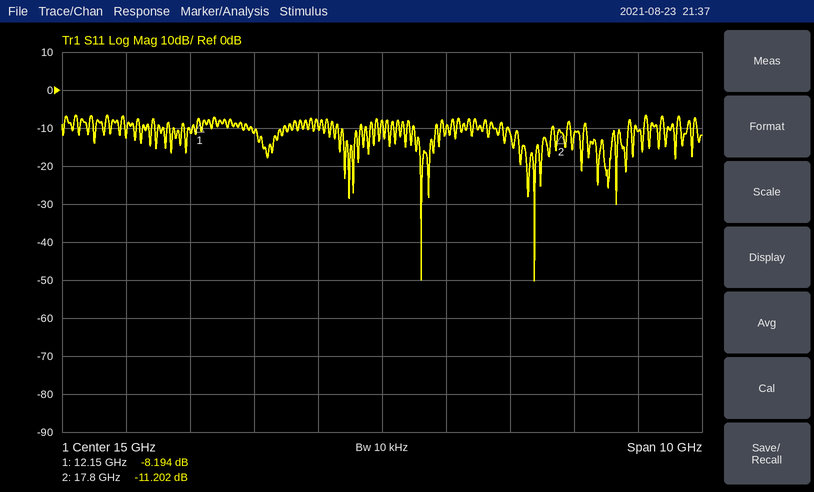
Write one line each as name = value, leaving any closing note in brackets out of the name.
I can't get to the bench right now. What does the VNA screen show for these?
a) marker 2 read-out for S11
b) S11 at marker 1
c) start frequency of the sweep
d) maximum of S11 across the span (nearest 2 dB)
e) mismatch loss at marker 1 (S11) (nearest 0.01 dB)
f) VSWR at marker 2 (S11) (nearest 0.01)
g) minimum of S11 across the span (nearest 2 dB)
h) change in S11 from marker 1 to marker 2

marker 2 read-out for S11 = -11.202 dB
S11 at marker 1 = -8.194 dB
start frequency of the sweep = 10 GHz
maximum of S11 across the span = -6 dB
mismatch loss at marker 1 (S11) = 0.71 dB
VSWR at marker 2 (S11) = 1.76
minimum of S11 across the span = -50 dB
change in S11 from marker 1 to marker 2 = -3.008 dB
